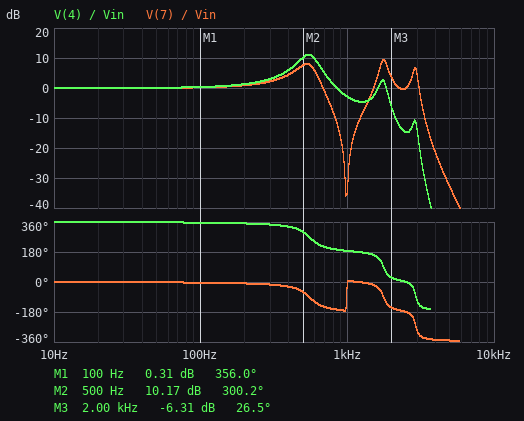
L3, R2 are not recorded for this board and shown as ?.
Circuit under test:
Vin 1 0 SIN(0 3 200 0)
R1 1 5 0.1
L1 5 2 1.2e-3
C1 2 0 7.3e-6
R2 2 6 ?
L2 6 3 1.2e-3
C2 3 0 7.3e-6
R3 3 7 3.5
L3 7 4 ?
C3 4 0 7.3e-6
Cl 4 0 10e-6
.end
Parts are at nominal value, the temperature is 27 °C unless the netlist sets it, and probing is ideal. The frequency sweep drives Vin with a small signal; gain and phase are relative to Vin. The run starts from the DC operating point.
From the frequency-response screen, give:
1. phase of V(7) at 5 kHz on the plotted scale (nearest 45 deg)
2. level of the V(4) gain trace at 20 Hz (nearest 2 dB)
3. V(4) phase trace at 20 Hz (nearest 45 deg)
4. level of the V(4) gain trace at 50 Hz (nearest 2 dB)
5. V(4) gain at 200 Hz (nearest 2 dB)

-360 deg
0 dB
360 deg
0 dB
2 dB
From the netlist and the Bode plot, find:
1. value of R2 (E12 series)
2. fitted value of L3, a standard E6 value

1.8 Ω
1.5 mH
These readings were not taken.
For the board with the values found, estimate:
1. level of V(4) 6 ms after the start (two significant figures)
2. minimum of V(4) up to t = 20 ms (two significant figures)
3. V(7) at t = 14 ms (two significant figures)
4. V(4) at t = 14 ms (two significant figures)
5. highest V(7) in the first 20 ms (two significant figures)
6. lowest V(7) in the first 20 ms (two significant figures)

3.1 V
-3.6 V
-3.3 V
-3.4 V
3.8 V
-3.4 V
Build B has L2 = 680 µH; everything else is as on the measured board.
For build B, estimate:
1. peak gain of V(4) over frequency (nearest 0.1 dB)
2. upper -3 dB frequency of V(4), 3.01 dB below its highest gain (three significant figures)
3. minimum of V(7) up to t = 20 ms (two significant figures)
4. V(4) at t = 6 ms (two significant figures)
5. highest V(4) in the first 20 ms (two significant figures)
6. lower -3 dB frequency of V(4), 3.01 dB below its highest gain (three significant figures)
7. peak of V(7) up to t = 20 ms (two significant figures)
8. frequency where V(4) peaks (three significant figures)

10.6 dB
691 Hz
-3.3 V
3.0 V
4.0 V
478 Hz
3.6 V
588 Hz
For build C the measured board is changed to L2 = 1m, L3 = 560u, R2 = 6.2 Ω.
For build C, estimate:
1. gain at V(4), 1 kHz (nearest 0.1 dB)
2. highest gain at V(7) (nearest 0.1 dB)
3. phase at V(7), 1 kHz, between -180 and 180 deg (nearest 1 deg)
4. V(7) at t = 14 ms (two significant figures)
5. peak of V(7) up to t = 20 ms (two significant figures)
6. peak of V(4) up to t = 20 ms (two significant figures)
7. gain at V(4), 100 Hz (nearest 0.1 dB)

-3.0 dB
2.9 dB
-154 deg
-3.2 V
3.3 V
3.4 V
0.2 dB
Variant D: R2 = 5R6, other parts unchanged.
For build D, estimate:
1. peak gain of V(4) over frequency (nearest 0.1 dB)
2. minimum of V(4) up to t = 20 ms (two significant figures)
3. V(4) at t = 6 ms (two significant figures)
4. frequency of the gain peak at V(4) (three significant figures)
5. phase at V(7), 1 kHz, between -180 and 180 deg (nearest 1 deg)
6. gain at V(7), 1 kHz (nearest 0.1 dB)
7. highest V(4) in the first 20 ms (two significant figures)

5.5 dB
-3.4 V
2.8 V
516 Hz
17 deg
-35.7 dB
3.6 V
